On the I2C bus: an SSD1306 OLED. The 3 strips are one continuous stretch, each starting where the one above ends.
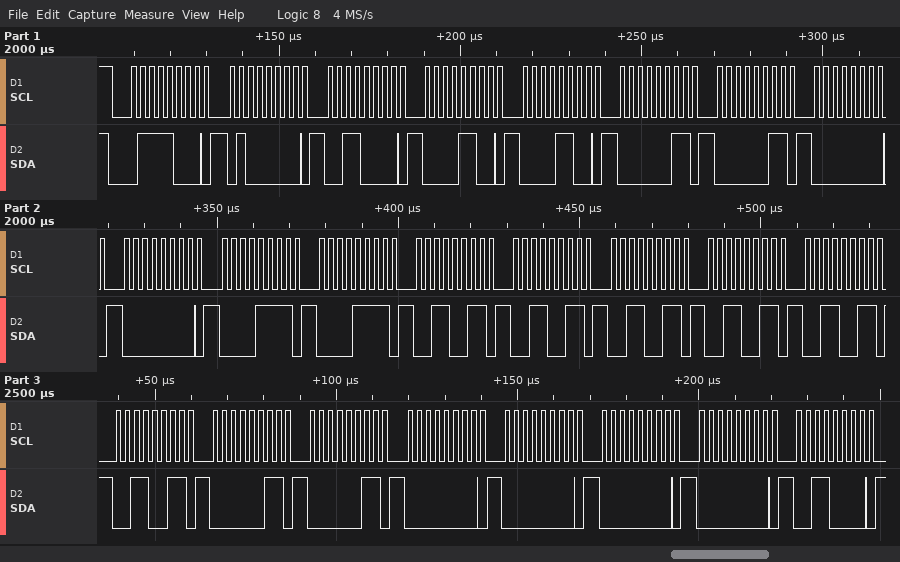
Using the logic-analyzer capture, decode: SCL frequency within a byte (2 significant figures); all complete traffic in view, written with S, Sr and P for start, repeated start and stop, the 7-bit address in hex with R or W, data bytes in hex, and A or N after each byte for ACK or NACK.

400 kHz
S 3CW A 40 A 30 A 0C A 0C A 03 A 03 A 00 A 00 A 0F A 0F A 33 A 33 A 33 A 33 A 33 A 33 A 03 A 03 A 00 A 00 A 00 A 00 A 30 A
